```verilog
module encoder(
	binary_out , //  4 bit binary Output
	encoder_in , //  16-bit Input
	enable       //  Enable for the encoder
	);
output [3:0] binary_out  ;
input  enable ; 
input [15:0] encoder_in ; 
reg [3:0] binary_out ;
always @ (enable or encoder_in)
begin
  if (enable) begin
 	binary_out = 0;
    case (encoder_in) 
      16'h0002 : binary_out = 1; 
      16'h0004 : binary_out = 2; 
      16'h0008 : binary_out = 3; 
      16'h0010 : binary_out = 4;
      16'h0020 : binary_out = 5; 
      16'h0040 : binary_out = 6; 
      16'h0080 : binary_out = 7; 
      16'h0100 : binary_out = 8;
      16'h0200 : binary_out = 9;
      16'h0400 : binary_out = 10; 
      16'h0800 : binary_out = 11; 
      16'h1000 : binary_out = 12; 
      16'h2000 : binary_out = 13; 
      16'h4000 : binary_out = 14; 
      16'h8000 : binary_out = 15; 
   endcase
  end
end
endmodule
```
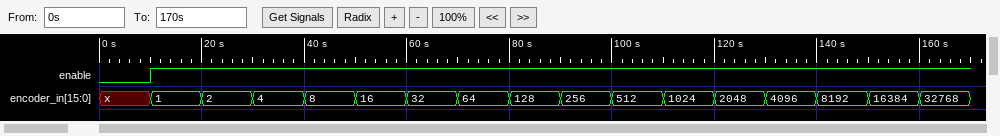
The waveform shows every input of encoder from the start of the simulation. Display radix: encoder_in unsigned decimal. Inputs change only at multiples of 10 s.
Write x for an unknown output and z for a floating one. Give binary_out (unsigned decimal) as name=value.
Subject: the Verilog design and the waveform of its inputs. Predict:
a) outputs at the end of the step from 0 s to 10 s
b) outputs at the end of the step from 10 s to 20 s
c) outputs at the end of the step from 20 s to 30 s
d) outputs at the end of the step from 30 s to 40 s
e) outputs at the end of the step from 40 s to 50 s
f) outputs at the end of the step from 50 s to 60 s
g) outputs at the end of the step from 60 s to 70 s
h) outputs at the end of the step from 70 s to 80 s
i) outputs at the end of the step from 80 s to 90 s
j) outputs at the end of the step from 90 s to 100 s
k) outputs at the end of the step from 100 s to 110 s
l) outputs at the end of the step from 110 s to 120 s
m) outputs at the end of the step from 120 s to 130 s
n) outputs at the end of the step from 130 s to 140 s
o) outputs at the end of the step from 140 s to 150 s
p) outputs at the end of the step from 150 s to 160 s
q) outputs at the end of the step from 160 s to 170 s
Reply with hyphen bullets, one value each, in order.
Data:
- binary_out=x
- binary_out=0
- binary_out=1
- binary_out=2
- binary_out=3
- binary_out=4
- binary_out=5
- binary_out=6
- binary_out=7
- binary_out=8
- binary_out=9
- binary_out=10
- binary_out=11
- binary_out=12
- binary_out=13
- binary_out=14
- binary_out=15
